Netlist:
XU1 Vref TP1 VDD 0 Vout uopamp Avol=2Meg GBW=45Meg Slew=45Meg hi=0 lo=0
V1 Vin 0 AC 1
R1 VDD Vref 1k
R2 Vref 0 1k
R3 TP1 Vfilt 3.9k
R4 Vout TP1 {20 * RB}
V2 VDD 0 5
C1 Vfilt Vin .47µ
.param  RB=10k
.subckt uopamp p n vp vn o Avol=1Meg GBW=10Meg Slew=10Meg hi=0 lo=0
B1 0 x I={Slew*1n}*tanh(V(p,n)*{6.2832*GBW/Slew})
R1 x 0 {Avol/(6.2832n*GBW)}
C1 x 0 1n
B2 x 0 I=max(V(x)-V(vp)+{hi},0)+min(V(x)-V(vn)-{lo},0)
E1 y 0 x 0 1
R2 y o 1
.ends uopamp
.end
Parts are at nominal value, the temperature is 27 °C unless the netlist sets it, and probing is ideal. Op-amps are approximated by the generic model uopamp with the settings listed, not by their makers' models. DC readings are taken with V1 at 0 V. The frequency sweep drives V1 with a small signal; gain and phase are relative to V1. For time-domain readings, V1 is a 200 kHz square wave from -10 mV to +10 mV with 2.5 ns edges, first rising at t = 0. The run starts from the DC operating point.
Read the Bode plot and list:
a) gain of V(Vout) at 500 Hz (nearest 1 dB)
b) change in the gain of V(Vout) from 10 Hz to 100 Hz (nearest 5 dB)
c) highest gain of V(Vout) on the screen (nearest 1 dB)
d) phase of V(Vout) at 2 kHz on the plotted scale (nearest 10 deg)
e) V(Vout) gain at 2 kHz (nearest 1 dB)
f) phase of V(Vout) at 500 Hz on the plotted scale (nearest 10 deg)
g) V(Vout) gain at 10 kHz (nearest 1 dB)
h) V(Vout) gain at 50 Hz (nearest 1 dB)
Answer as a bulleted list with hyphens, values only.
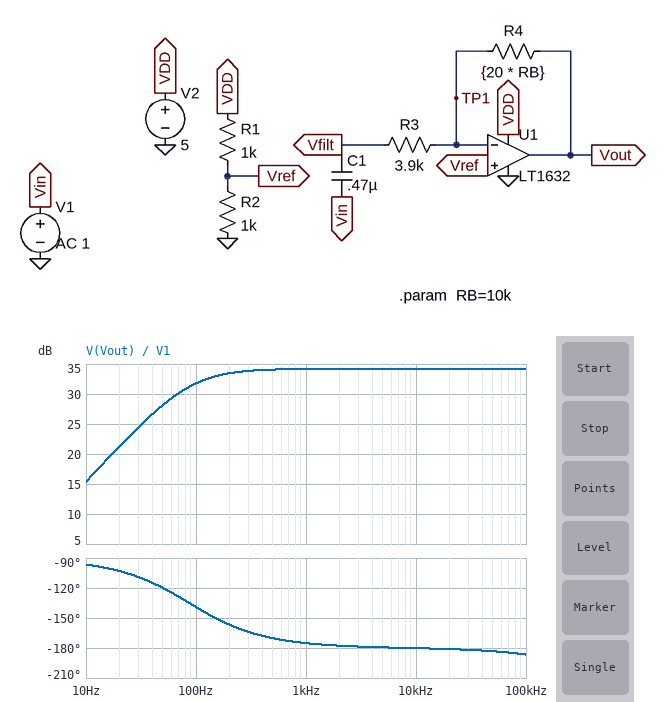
- 34 dB
- 15 dB
- 34 dB
- -180 deg
- 34 dB
- -170 deg
- 34 dB
- 28 dB
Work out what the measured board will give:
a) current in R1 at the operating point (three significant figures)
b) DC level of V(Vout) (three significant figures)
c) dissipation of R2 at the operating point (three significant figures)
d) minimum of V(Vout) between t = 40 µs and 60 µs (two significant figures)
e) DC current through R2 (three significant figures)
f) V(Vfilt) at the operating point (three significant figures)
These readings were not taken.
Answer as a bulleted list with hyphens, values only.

- 2.50 mA
- 2.50 V
- 6.25 mW
- 1.5 V
- 2.50 mA
- 2.50 V
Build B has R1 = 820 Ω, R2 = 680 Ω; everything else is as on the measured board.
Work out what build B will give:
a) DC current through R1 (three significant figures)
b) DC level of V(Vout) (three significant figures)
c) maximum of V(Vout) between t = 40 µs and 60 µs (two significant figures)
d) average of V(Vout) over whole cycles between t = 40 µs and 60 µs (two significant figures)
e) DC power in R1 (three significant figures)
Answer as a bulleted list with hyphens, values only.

- 3.33 mA
- 2.27 V
- 2.3 V
- 1.8 V
- 9.11 mW
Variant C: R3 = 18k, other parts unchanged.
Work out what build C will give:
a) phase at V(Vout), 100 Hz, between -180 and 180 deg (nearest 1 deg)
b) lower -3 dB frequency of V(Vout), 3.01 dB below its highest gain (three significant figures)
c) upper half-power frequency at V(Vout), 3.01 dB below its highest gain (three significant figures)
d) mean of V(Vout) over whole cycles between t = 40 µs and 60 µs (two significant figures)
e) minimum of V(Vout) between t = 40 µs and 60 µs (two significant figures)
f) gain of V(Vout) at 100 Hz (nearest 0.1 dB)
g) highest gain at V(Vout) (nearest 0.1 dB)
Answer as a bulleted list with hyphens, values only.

- -169 deg
- 18.8 Hz
- 3.72 MHz
- 2.4 V
- 2.3 V
- 20.8 dB
- 20.9 dB
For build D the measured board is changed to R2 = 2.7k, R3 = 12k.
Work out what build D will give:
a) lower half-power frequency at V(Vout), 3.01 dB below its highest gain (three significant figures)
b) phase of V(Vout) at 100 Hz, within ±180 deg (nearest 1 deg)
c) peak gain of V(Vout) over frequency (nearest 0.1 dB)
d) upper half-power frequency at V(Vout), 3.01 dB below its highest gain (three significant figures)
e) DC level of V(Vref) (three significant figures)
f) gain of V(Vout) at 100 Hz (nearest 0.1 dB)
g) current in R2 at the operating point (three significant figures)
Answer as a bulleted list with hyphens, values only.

- 28.2 Hz
- -164 deg
- 24.4 dB
- 2.55 MHz
- 3.65 V
- 24.1 dB
- 1.35 mA
